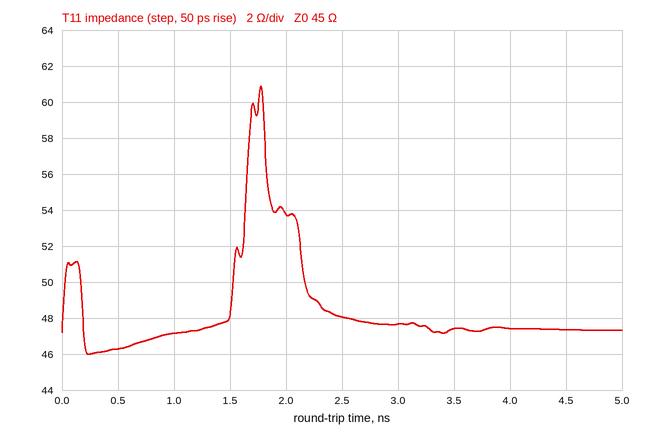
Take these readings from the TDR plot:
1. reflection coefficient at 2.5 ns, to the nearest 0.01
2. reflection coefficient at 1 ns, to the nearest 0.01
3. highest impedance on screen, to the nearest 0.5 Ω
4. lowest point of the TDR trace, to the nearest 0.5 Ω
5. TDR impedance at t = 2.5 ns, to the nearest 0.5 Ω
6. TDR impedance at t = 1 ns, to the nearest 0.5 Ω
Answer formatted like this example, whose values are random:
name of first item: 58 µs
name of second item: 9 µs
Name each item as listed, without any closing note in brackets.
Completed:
reflection coefficient at 2.5 ns, to the nearest 0.01: +0.03
reflection coefficient at 1 ns, to the nearest 0.01: +0.02
highest impedance on screen, to the nearest 0.5 Ω: 61.0 Ω
lowest point of the TDR trace, to the nearest 0.5 Ω: 46.0 Ω
TDR impedance at t = 2.5 ns, to the nearest 0.5 Ω: 48.0 Ω
TDR impedance at t = 1 ns, to the nearest 0.5 Ω: 47.0 Ω
